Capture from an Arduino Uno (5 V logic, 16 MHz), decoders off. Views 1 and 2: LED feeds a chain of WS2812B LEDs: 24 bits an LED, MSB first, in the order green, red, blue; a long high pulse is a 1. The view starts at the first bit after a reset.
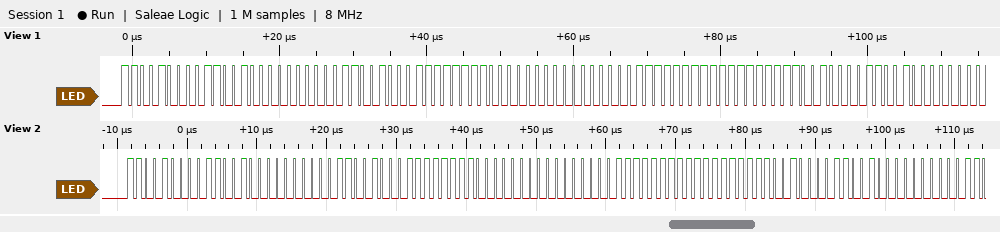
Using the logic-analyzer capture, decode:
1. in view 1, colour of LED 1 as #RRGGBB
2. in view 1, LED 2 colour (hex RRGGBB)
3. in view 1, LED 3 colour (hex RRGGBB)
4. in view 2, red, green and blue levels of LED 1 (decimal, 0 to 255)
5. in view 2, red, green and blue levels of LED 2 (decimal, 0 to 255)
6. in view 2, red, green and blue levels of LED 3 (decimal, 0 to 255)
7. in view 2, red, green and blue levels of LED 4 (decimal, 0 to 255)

#64C800
#FFC800
#FF00FF
100, 200, 0
255, 200, 0
255, 0, 255
100, 200, 0
